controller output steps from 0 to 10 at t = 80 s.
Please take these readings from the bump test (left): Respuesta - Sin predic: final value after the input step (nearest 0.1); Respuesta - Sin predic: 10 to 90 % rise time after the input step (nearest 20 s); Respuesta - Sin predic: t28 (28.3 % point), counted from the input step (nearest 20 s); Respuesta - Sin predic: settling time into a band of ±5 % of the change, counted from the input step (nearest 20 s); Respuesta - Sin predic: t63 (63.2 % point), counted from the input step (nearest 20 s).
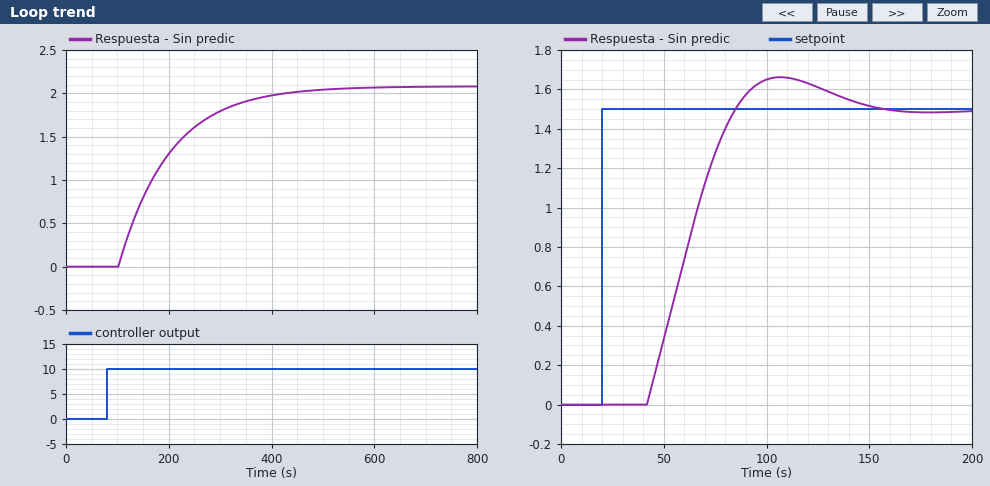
2.1
220 s
60 s
320 s
120 s
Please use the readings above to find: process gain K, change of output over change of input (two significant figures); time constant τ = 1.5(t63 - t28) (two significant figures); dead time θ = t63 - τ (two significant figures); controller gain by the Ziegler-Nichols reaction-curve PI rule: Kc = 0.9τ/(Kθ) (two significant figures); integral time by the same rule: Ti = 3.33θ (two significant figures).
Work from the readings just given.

0.21
90 s
30 s
13
100 s
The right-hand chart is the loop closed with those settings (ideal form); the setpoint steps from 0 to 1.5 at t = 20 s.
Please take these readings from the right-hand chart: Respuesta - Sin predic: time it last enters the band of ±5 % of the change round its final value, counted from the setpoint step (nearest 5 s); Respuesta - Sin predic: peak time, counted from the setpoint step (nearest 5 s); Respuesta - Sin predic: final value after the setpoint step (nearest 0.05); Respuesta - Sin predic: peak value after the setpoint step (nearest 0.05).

115 s
85 s
1.50
1.65
